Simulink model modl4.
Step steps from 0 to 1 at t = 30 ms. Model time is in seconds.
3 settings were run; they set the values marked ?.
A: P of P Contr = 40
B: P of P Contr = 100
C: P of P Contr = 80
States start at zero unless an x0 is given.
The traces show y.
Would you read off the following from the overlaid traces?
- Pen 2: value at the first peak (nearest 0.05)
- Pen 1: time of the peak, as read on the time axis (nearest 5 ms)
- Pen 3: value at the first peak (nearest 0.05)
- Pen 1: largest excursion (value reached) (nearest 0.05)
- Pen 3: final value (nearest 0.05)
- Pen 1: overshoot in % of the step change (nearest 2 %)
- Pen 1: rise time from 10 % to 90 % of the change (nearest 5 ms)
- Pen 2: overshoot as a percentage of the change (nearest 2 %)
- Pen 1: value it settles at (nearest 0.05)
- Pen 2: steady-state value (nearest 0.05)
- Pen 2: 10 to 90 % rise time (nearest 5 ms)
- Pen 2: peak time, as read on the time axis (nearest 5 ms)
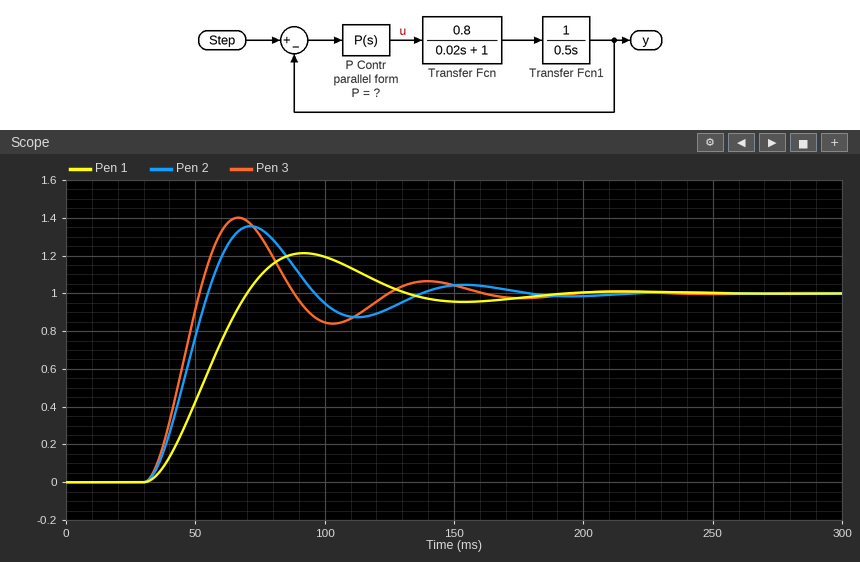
1.35
90 ms
1.40
1.20
1.00
22 %
25 ms
36 %
1.00
1.00
15 ms
70 ms
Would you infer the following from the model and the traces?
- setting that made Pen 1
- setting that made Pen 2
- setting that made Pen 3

A
C
B
